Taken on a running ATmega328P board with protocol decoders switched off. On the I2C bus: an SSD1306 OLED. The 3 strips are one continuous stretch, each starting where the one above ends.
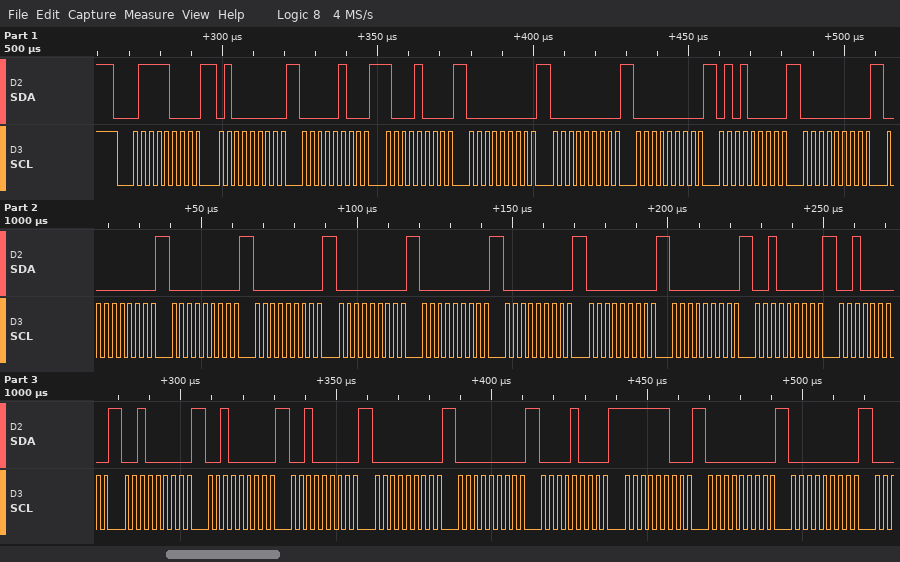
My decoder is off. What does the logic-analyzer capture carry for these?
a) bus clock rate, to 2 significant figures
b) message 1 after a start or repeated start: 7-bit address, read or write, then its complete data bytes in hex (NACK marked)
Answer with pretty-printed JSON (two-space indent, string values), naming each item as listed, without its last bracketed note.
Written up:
{
  "bus clock rate, to 2 significant figures": "400 kHz",
  "message 1 after a start or repeated start: 7-bit address, read or write, then its complete data bytes in hex": "0x3C write: 40 04 88 00 00 00 50 00 00 00 00 00 00 00 00 00 20 20 20 20 20 00 00 08 FC 00 00"
}
